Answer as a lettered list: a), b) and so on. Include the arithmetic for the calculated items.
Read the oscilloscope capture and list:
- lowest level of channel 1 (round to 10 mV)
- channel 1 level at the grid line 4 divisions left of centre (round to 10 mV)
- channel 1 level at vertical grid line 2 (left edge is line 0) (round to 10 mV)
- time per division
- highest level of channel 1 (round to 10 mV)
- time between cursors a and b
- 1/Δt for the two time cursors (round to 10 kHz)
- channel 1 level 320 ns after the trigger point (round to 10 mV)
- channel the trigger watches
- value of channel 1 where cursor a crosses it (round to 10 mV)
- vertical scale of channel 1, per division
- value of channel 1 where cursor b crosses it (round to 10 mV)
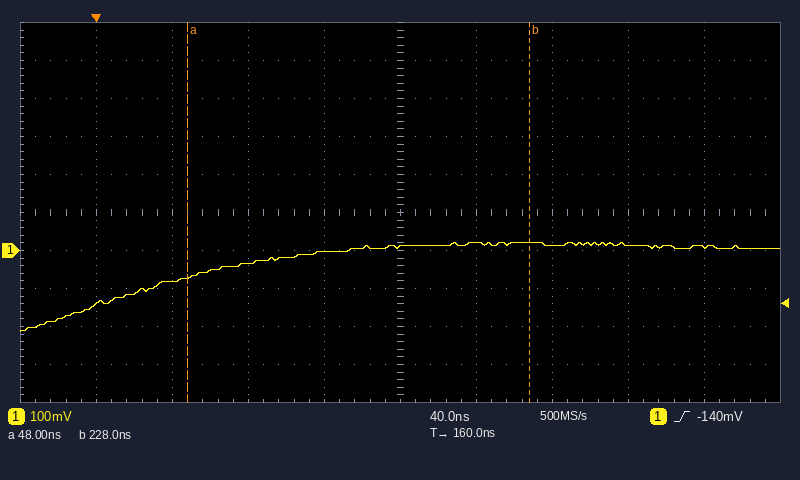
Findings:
a) -210 mV
b) -140 mV
c) -80 mV
d) 40 ns
e) 20 mV
f) 228 ns − (48 ns) = 180 ns
g) 1 / 180 ns ≈ 5.56 MHz
h) 10 mV
i) channel 1
j) -70 mV
k) 100 mV
l) 20 mV
